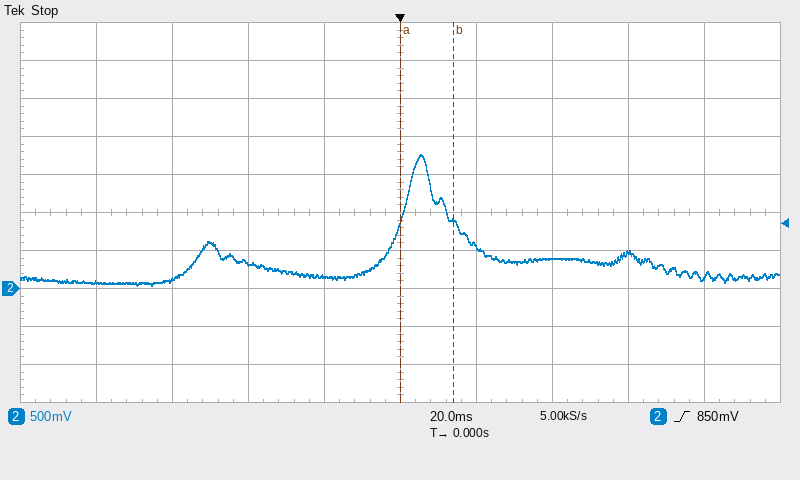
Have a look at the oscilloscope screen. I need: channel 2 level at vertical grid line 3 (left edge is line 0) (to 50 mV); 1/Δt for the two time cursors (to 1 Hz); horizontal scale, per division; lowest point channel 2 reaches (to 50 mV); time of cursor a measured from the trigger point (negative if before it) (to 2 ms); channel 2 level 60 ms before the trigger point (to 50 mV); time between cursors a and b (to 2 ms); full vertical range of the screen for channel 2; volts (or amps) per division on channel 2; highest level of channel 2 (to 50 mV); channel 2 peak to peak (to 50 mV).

350 mV
71 Hz
20 ms
50 mV
0 ms
100 mV
14 ms
5 V
500 mV
1.75 V
1.70 V
